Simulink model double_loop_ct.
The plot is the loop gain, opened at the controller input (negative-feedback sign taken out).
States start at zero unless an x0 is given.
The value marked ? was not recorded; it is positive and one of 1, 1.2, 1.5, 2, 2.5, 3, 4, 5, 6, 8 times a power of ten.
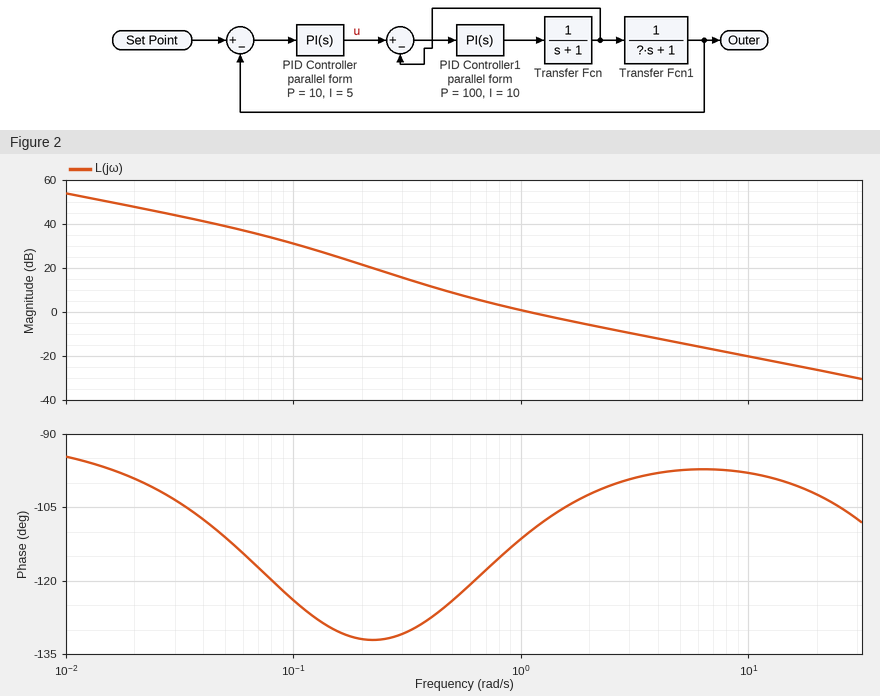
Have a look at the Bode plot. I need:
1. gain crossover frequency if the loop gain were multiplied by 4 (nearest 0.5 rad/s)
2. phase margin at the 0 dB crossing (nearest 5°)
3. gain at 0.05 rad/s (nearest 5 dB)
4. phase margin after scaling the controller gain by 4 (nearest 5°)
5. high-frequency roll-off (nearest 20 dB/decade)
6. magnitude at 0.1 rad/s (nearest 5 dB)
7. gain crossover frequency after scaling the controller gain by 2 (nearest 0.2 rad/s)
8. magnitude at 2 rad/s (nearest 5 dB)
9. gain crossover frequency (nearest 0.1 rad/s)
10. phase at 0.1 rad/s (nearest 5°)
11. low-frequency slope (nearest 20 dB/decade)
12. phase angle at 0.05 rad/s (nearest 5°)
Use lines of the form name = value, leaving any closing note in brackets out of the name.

gain crossover frequency if the loop gain were multiplied by 4 = 4.0 rad/s
phase margin at the 0 dB crossing = 70°
gain at 0.05 rad/s = 40 dB
phase margin after scaling the controller gain by 4 = 80°
high-frequency roll-off = -20 dB/decade
magnitude at 0.1 rad/s = 30 dB
gain crossover frequency after scaling the controller gain by 2 = 2.0 rad/s
magnitude at 2 rad/s = -5 dB
gain crossover frequency = 1.1 rad/s
phase at 0.1 rad/s = -125°
low-frequency slope = -20 dB/decade
phase angle at 0.05 rad/s = -110°
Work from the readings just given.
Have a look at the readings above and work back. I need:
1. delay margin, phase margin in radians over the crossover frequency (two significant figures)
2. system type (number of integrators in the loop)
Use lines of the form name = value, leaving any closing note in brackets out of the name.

delay margin, phase margin in radians over the crossover frequency = 1.1 s
system type = 1
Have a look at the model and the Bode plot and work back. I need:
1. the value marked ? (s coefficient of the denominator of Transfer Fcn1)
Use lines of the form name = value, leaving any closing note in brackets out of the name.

the value marked ? = 10
